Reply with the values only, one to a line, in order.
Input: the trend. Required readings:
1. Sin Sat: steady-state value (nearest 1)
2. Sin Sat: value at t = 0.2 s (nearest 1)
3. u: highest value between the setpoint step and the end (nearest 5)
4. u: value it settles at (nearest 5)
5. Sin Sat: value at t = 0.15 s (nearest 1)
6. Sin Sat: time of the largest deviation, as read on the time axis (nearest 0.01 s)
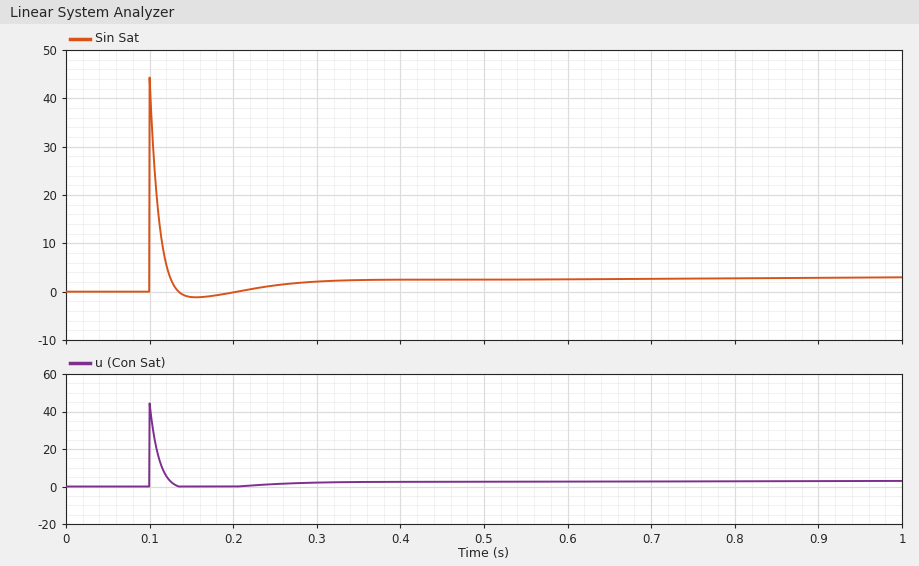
3
0
45
5
-1
0.10 s
